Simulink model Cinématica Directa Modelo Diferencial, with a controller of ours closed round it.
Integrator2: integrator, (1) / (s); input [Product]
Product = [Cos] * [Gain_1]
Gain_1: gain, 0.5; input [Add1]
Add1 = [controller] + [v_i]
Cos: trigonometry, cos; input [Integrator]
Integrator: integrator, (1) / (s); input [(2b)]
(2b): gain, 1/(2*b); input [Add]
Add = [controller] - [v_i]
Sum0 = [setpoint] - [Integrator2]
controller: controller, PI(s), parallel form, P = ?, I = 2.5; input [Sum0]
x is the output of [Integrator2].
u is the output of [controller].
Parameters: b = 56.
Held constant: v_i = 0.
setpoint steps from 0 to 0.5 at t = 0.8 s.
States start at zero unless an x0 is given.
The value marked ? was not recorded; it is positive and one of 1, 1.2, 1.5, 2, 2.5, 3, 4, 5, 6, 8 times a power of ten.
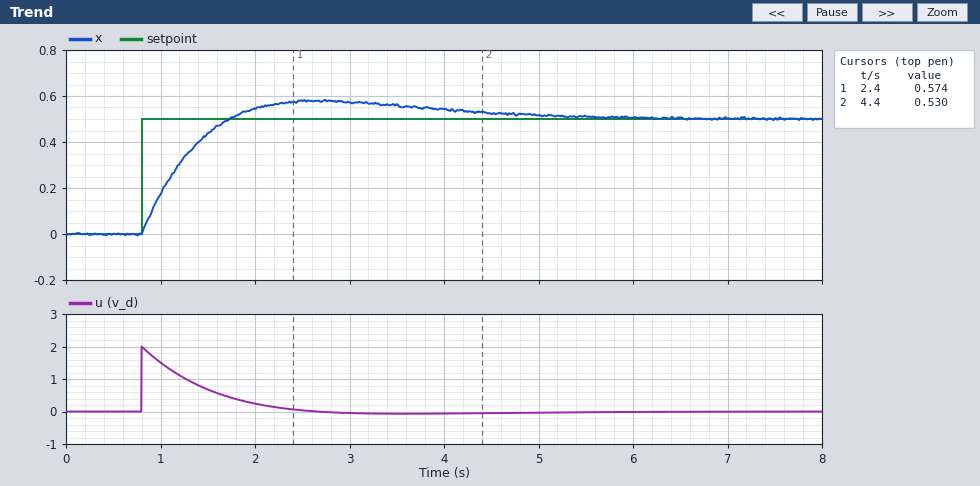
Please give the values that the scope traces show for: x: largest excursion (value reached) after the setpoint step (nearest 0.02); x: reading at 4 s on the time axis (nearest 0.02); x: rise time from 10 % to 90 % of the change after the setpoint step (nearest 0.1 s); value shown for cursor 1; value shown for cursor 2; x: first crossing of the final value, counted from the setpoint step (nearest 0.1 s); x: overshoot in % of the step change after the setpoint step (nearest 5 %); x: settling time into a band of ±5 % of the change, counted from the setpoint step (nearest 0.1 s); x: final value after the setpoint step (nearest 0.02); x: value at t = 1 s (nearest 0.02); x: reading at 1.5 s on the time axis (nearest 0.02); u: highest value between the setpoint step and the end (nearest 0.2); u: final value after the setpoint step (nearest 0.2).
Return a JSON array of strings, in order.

["0.58", "0.54", "0.7 s", "0.574", "0.530", "0.9 s", "15 %", "3.8 s", "0.50", "0.18", "0.44", "2.0", "0.0"]
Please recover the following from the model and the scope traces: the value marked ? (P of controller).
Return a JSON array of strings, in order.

["4"]
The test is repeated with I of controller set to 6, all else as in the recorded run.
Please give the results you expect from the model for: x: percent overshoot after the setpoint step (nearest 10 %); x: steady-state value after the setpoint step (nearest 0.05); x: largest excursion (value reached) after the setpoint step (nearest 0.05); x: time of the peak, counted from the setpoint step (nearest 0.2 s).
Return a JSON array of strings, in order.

["30 %", "0.50", "0.65", "1.4 s"]
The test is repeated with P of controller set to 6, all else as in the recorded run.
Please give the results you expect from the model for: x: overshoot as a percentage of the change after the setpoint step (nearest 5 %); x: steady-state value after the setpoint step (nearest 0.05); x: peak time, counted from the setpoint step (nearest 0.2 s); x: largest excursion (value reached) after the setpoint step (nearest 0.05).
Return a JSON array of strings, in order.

["10 %", "0.50", "1.6 s", "0.55"]
